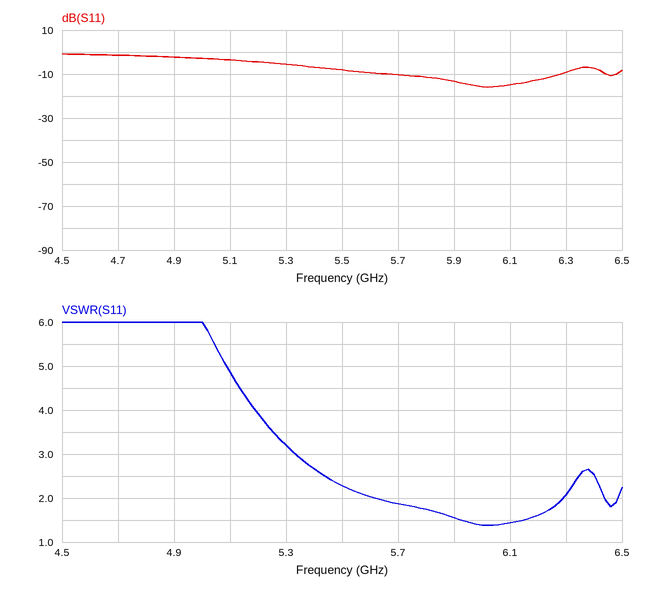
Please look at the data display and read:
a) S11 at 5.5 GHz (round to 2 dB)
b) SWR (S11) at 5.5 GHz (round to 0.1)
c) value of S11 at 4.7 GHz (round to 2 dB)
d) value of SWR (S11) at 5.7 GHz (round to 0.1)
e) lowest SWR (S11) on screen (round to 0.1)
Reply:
-8 dB
2.3
-2 dB
1.9
1.4
